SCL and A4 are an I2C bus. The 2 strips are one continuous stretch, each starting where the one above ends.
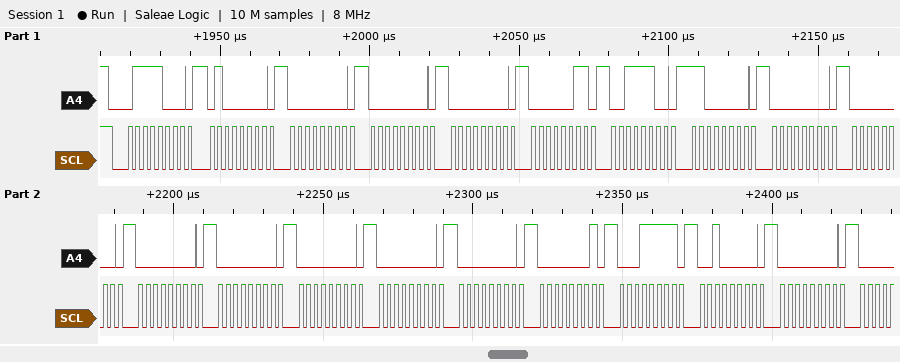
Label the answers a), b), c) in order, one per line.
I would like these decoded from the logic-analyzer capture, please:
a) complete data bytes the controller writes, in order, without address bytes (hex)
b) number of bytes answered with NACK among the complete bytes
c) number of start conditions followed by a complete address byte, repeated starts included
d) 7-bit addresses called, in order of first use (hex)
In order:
a) 40 00 00 00 03 3C C0 00 00 00 00 00 00 00 01 1F 20 00
b) 0
c) 1
d) 0x3C
